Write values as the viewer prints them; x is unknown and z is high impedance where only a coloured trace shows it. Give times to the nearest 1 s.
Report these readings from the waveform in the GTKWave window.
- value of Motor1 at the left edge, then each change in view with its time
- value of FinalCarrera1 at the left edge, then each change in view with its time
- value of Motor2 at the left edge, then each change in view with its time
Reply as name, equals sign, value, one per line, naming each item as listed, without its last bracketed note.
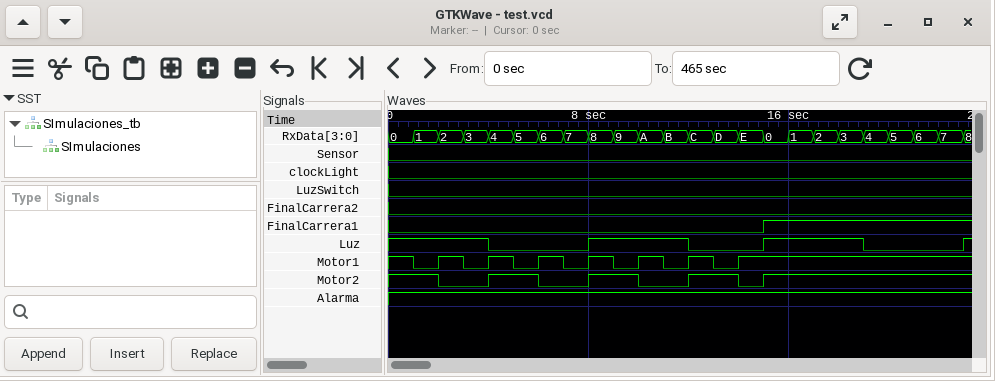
value of Motor1 at the left edge, then each change in view with its time = 1, 0 at 1 s, 1 at 2 s, 0 at 3 s, 1 at 4 s, 0 at 5 s, 1 at 6 s, 0 at 7 s, 1 at 8 s, 0 at 9 s, 1 at 10 s, 0 at 11 s, 1 at 12 s, 0 at 13 s, 1 at 14 s
value of FinalCarrera1 at the left edge, then each change in view with its time = 0, 1 at 15 s
value of Motor2 at the left edge, then each change in view with its time = 1, 0 at 2 s, 1 at 4 s, 0 at 6 s, 1 at 8 s, 0 at 10 s, 1 at 12 s, 0 at 14 s, 1 at 15 s
